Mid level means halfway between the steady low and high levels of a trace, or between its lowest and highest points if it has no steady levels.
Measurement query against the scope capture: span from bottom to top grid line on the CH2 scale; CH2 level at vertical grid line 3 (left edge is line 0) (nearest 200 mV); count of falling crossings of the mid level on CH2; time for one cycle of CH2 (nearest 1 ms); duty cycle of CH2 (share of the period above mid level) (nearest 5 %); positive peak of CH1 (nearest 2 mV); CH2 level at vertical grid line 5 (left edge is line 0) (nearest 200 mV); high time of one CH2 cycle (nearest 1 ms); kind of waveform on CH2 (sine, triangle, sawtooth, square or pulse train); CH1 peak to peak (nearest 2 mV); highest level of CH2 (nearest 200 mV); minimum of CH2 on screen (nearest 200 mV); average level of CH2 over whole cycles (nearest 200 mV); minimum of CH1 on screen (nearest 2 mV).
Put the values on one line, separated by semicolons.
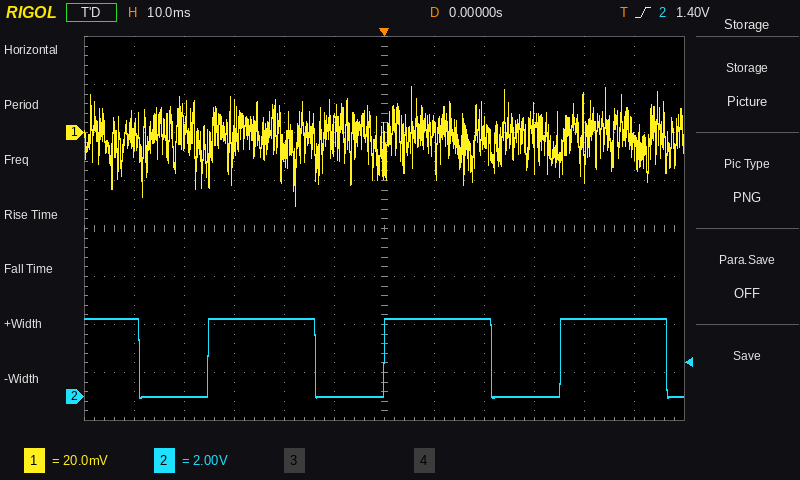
16 V; 3.2 V; 4; 35 ms; 60 %; 20 mV; 0.0 V; 21 ms; pulse train; 50 mV; 3.2 V; 0.0 V; 2.0 V; -30 mV
